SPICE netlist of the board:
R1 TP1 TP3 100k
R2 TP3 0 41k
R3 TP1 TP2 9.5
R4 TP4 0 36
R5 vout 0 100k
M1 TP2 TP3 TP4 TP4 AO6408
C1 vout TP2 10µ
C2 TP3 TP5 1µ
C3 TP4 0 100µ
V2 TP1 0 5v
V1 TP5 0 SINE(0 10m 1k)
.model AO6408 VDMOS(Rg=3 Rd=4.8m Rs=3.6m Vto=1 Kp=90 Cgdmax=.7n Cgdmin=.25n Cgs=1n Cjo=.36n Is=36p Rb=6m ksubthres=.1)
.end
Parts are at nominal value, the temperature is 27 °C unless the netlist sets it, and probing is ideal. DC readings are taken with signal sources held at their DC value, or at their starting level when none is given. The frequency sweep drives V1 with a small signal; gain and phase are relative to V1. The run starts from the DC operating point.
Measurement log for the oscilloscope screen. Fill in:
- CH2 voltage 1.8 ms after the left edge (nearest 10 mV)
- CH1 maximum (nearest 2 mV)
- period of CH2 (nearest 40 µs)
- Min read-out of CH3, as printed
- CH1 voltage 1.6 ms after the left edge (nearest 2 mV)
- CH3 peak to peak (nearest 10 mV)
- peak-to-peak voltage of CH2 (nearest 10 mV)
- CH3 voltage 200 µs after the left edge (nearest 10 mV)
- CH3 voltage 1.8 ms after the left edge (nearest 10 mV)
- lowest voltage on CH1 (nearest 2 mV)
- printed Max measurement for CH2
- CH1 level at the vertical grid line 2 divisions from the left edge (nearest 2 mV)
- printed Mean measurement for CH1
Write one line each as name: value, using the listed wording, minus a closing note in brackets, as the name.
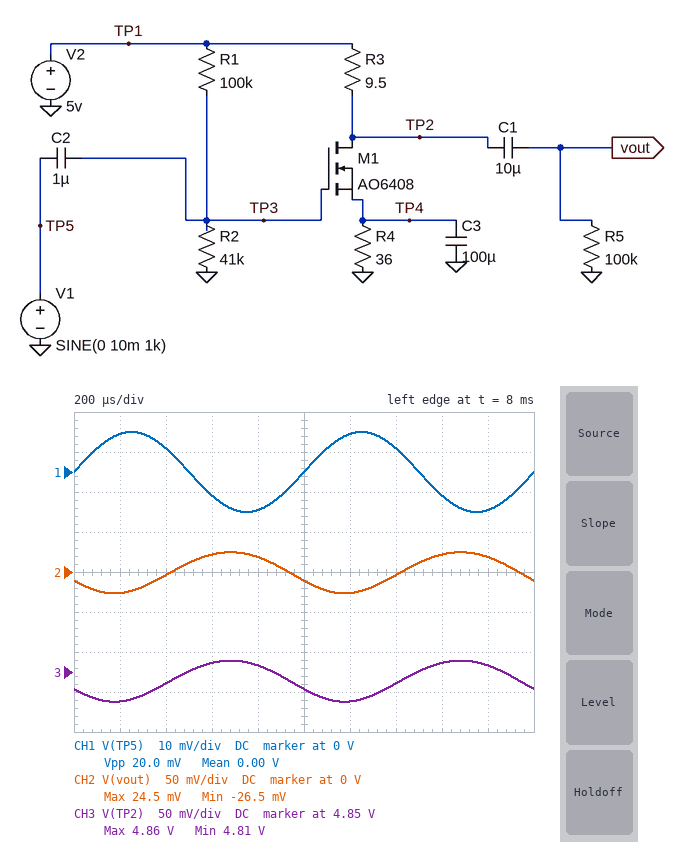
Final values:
CH2 voltage 1.8 ms after the left edge: 20 mV
CH1 maximum: 10 mV
period of CH2: 1.00 ms
Min read-out of CH3, as printed: 4.81 V
CH1 voltage 1.6 ms after the left edge: -6 mV
CH3 peak to peak: 50 mV
peak-to-peak voltage of CH2: 50 mV
CH3 voltage 200 µs after the left edge: 4.81 V
CH3 voltage 1.8 ms after the left edge: 4.86 V
lowest voltage on CH1: -10 mV
printed Max measurement for CH2: 24.5 mV
CH1 level at the vertical grid line 2 divisions from the left edge: 6 mV
printed Mean measurement for CH1: 0.00 V
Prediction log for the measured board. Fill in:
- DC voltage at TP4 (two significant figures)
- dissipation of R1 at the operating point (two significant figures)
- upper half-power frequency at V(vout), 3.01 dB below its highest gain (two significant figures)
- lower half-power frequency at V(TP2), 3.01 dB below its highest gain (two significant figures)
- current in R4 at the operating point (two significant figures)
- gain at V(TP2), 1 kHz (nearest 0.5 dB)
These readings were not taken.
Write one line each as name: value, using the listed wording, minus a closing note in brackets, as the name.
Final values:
DC voltage at TP4: 610 mV
dissipation of R1 at the operating point: 130 µW
upper half-power frequency at V(vout), 3.01 dB below its highest gain: 17 MHz
lower half-power frequency at V(TP2), 3.01 dB below its highest gain: 530 Hz
current in R4 at the operating point: 17 mA
gain at V(TP2), 1 kHz: 8.0 dB
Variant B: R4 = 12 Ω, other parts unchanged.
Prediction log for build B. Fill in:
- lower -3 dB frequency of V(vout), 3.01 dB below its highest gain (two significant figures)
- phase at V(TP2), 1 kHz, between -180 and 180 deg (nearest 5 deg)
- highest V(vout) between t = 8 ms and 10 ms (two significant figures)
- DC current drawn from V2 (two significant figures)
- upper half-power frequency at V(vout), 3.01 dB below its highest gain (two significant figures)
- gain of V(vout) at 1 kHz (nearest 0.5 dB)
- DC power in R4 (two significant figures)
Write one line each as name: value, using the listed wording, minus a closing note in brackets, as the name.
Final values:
lower -3 dB frequency of V(vout), 3.01 dB below its highest gain: 1.4 kHz
phase at V(TP2), 1 kHz, between -180 and 180 deg: -135 deg
highest V(vout) between t = 8 ms and 10 ms: 43 mV
DC current drawn from V2: 46 mA
upper half-power frequency at V(vout), 3.01 dB below its highest gain: 11 MHz
gain of V(vout) at 1 kHz: 13.0 dB
DC power in R4: 25 mW
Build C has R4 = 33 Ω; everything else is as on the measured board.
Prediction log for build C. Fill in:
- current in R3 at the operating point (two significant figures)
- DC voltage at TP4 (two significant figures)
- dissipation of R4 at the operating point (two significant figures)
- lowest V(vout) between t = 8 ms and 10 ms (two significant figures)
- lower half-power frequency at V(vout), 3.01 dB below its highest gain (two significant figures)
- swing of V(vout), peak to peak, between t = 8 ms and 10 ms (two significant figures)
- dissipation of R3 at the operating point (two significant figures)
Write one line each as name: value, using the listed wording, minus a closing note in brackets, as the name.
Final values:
current in R3 at the operating point: 18 mA
DC voltage at TP4: 600 mV
dissipation of R4 at the operating point: 11 mW
lowest V(vout) between t = 8 ms and 10 ms: -28 mV
lower half-power frequency at V(vout), 3.01 dB below its highest gain: 570 Hz
swing of V(vout), peak to peak, between t = 8 ms and 10 ms: 54 mV
dissipation of R3 at the operating point: 3.2 mW
